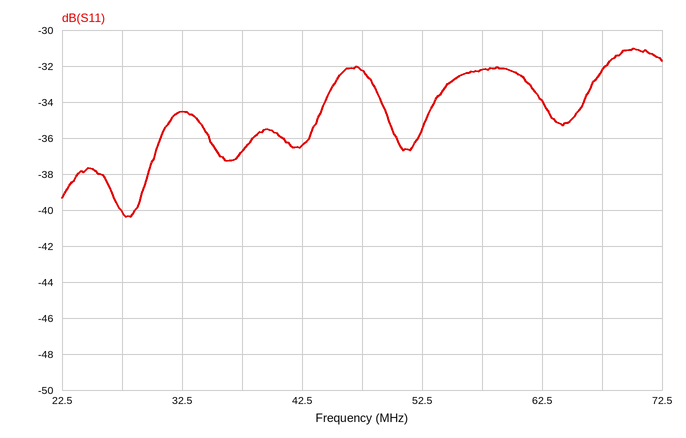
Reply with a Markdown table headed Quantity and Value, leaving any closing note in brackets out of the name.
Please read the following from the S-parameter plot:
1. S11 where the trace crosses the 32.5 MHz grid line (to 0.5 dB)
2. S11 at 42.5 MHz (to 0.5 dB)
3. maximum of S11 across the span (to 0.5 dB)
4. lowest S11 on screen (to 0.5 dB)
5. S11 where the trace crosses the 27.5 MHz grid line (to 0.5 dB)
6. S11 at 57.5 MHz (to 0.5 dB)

| Quantity | Value |
|---|---|
| S11 where the trace crosses the 32.5 MHz grid line | -34.5 dB |
| S11 at 42.5 MHz | -36.5 dB |
| maximum of S11 across the span | -31.0 dB |
| lowest S11 on screen | -40.5 dB |
| S11 where the trace crosses the 27.5 MHz grid line | -40.0 dB |
| S11 at 57.5 MHz | -32.0 dB |
